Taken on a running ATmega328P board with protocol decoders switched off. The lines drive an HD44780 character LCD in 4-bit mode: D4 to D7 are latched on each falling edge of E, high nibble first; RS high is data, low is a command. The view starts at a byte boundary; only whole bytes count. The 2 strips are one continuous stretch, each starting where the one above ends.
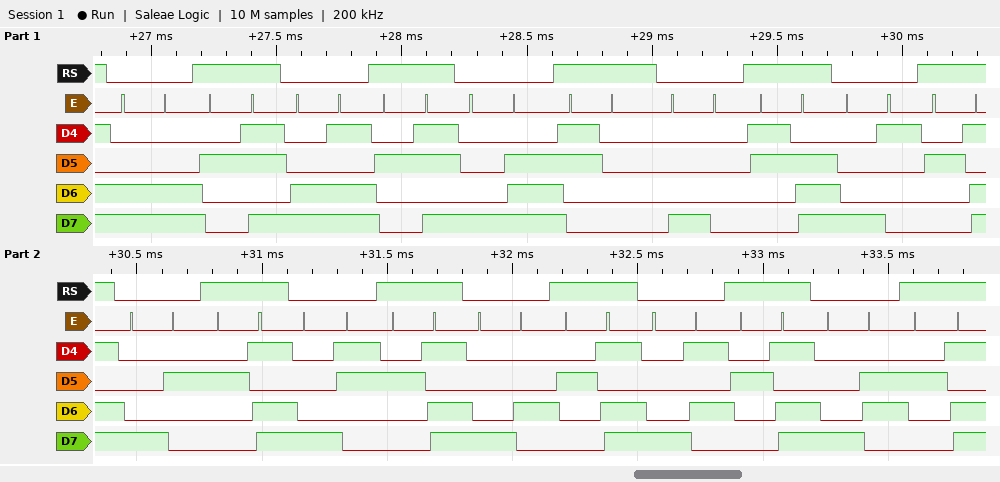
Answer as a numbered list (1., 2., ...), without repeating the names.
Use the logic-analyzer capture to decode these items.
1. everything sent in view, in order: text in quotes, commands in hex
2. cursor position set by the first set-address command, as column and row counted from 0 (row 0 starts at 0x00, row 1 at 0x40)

1. 0xCC "+" 0xCD "+" 0x8E "0" 0x80 ">" 0x81 "-" 0x82 "-" 0x83 "-" 0x84 "-" 0x85 "-" 0x86 "-"
2. column 12, row 1
